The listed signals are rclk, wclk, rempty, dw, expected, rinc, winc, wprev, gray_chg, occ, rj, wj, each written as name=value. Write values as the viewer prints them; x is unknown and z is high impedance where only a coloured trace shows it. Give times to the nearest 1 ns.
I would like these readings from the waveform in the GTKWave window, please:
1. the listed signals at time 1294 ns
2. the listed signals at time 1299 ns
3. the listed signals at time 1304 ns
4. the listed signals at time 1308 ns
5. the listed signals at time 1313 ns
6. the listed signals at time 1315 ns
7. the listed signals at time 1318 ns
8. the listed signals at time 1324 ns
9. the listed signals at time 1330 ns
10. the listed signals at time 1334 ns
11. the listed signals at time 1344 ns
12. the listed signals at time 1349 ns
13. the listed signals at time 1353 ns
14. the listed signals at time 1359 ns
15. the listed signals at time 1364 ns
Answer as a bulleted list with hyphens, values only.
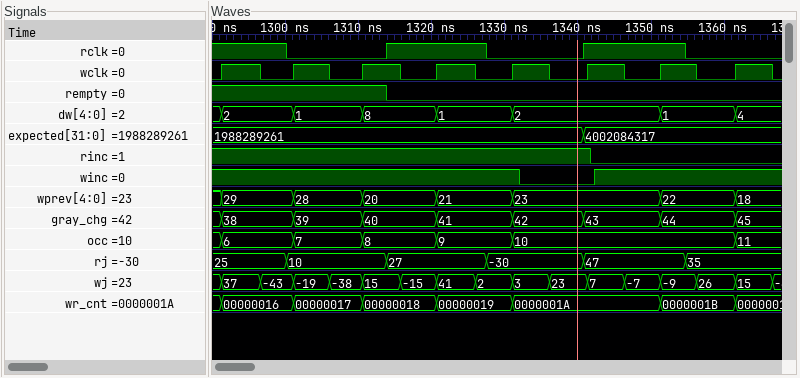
- rclk=1, wclk=1, rempty=1, dw=2, expected=1988289261, rinc=1, winc=1, wprev=29, gray_chg=38, occ=6, rj=25, wj=37
- rclk=1, wclk=0, rempty=1, dw=2, expected=1988289261, rinc=1, winc=1, wprev=29, gray_chg=38, occ=6, rj=25, wj=-43
- rclk=0, wclk=1, rempty=1, dw=1, expected=1988289261, rinc=1, winc=1, wprev=28, gray_chg=39, occ=7, rj=10, wj=-19
- rclk=0, wclk=0, rempty=1, dw=1, expected=1988289261, rinc=1, winc=1, wprev=28, gray_chg=39, occ=7, rj=10, wj=-38
- rclk=0, wclk=1, rempty=1, dw=8, expected=1988289261, rinc=1, winc=1, wprev=20, gray_chg=40, occ=8, rj=10, wj=15
- rclk=1, wclk=1, rempty=0, dw=8, expected=1988289261, rinc=1, winc=1, wprev=20, gray_chg=40, occ=8, rj=27, wj=15
- rclk=1, wclk=0, rempty=0, dw=8, expected=1988289261, rinc=1, winc=1, wprev=20, gray_chg=40, occ=8, rj=27, wj=-15
- rclk=1, wclk=1, rempty=0, dw=1, expected=1988289261, rinc=1, winc=1, wprev=21, gray_chg=41, occ=9, rj=27, wj=41
- rclk=0, wclk=0, rempty=0, dw=1, expected=1988289261, rinc=1, winc=1, wprev=21, gray_chg=41, occ=9, rj=-30, wj=2
- rclk=0, wclk=1, rempty=0, dw=2, expected=1988289261, rinc=1, winc=0, wprev=23, gray_chg=42, occ=10, rj=-30, wj=3
- rclk=1, wclk=1, rempty=0, dw=2, expected=4002084317, rinc=0, winc=1, wprev=23, gray_chg=43, occ=10, rj=47, wj=7
- rclk=1, wclk=0, rempty=0, dw=2, expected=4002084317, rinc=0, winc=1, wprev=23, gray_chg=43, occ=10, rj=47, wj=-7
- rclk=1, wclk=1, rempty=0, dw=1, expected=4002084317, rinc=0, winc=1, wprev=22, gray_chg=44, occ=10, rj=47, wj=-9
- rclk=0, wclk=0, rempty=0, dw=1, expected=4002084317, rinc=0, winc=1, wprev=22, gray_chg=44, occ=10, rj=35, wj=26
- rclk=0, wclk=1, rempty=0, dw=4, expected=4002084317, rinc=0, winc=1, wprev=18, gray_chg=45, occ=11, rj=35, wj=15
